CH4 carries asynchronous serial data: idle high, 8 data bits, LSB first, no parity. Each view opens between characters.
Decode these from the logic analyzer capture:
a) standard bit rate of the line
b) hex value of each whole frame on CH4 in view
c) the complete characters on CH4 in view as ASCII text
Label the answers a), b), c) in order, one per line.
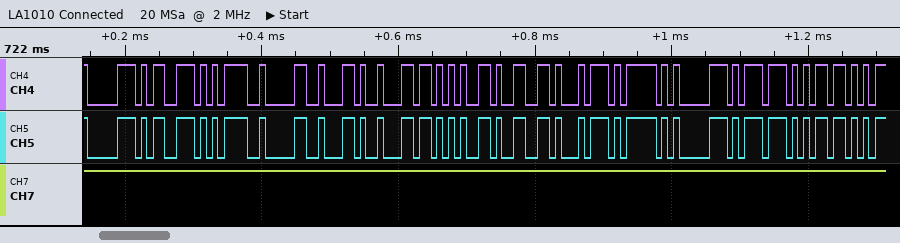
a) 115200 baud
b) 70, 73, 3D, 30, 2C, 6C, 65, 66, 74, 5F, 70, 77, 6D
c) "ps=0,left_pwm"
